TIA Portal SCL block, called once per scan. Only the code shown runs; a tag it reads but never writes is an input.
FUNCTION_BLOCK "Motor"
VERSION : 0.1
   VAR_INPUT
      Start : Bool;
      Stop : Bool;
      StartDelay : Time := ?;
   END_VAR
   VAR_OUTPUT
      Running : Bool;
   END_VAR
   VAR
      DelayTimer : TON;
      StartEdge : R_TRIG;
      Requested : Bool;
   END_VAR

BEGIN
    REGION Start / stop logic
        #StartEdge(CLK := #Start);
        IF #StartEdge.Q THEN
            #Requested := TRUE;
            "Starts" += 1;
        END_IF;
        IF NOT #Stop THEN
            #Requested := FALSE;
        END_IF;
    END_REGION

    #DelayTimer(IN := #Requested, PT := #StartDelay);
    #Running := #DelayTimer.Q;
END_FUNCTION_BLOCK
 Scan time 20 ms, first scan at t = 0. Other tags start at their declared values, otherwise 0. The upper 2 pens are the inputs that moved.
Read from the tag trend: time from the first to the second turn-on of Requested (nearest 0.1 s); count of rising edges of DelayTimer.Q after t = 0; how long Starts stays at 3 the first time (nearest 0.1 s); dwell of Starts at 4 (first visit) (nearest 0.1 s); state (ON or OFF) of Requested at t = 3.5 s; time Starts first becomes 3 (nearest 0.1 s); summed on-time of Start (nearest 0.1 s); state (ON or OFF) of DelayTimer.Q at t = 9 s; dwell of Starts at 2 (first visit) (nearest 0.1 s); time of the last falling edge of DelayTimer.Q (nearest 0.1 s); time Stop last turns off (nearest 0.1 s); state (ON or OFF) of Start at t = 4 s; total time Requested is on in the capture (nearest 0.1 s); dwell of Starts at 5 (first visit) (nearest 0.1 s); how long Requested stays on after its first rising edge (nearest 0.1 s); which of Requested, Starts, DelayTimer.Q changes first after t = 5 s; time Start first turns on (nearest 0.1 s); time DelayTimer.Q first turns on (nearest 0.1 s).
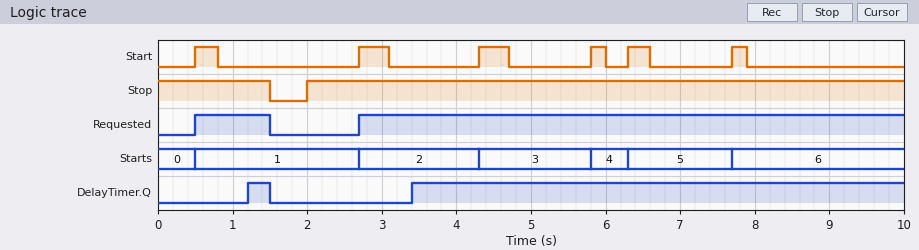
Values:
2.2 s
2
1.5 s
0.5 s
ON
4.3 s
1.8 s
ON
1.6 s
1.5 s
1.5 s
OFF
8.3 s
1.4 s
1.0 s
Starts
0.5 s
1.2 s
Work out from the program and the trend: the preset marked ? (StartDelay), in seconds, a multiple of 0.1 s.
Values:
0.7 s
